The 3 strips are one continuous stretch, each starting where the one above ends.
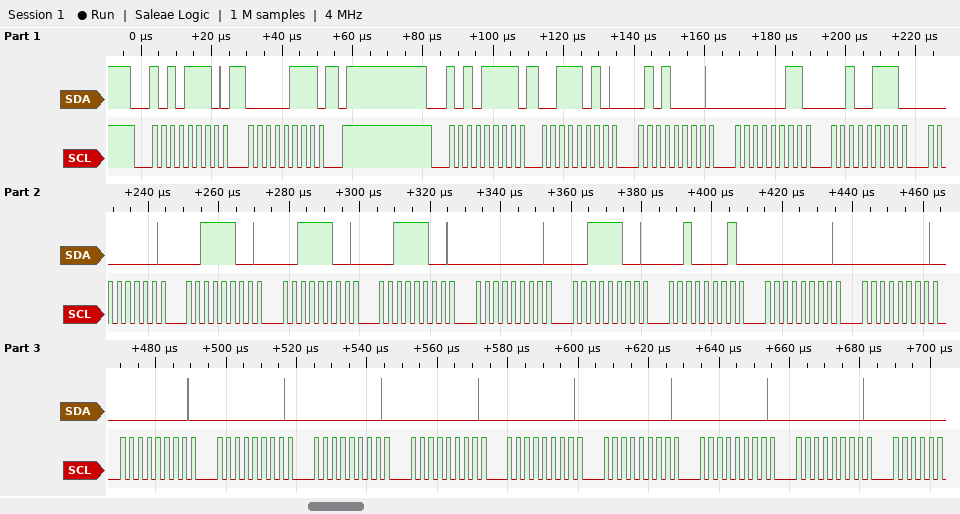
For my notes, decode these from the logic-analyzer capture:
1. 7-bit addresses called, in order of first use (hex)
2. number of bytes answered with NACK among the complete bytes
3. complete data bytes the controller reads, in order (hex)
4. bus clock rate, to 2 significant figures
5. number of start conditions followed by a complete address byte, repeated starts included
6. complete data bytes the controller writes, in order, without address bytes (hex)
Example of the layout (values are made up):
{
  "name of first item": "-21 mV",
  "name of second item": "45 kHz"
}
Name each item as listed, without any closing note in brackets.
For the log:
{
  "7-bit addresses called, in order of first use": "0x57",
  "number of bytes answered with NACK among the complete bytes": "0",
  "complete data bytes the controller reads, in order": "3A 50 03 27 00 3C 3C 3C 00 3C 21 00 00 00 00 00 00 00 00 00 00",
  "bus clock rate, to 2 significant figures": "400 kHz",
  "number of start conditions followed by a complete address byte, repeated starts included": "2",
  "complete data bytes the controller writes, in order, without address bytes": "07"
}
